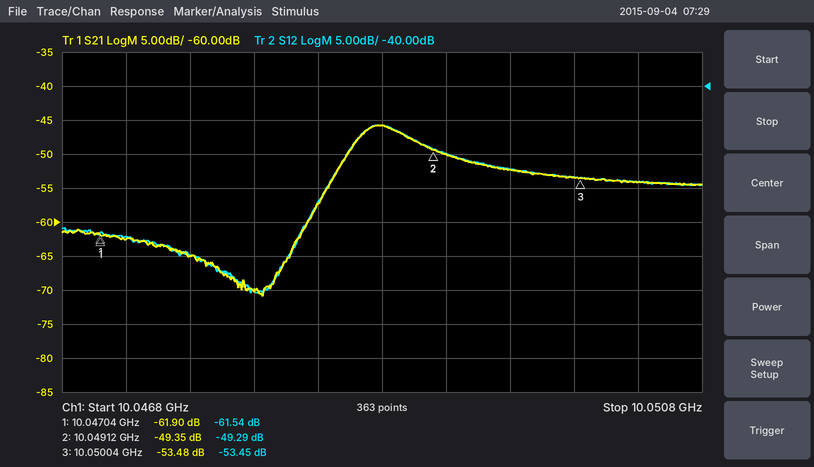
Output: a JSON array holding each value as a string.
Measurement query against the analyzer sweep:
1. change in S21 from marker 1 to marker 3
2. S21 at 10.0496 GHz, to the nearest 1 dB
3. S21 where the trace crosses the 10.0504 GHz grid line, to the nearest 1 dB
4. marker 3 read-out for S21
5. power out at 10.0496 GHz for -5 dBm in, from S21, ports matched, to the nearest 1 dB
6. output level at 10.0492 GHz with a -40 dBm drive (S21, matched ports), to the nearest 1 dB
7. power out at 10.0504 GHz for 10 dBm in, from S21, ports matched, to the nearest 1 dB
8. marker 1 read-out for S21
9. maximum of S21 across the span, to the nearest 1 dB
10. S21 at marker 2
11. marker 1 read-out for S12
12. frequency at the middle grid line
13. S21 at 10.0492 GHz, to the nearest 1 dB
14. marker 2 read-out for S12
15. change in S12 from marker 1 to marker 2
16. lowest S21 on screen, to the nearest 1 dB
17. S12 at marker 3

["8.42 dB", "-52 dB", "-54 dB", "-53.48 dB", "-57 dBm", "-90 dBm", "-44 dBm", "-61.90 dB", "-46 dB", "-49.35 dB", "-61.54 dB", "10.0488 GHz", "-50 dB", "-49.29 dB", "12.25 dB", "-71 dB", "-53.45 dB"]
